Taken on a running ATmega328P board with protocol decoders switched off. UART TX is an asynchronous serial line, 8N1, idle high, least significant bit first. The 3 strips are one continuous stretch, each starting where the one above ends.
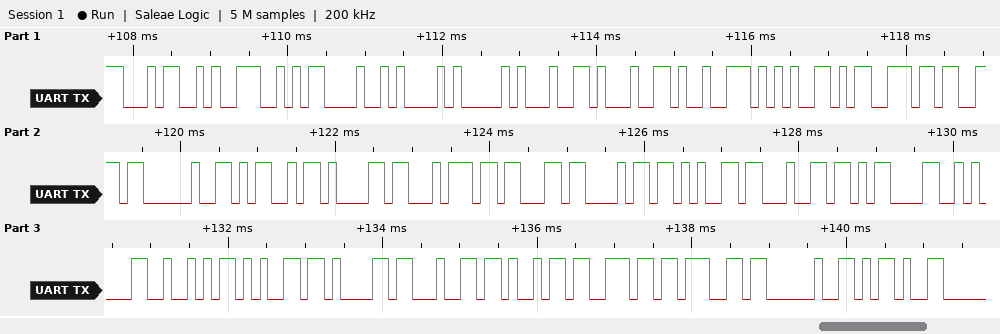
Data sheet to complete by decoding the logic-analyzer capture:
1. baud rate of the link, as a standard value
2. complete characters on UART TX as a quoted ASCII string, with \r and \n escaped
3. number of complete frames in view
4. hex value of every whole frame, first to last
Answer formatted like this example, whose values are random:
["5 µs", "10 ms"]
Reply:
["9600 baud", "\"49\\r\\nAddress Matched\\r\\nReading -\"", "30", "34 39 0D 0A 41 64 64 72 65 73 73 20 4D 61 74 63 68 65 64 0D 0A 52 65 61 64 69 6E 67 20 2D"]
